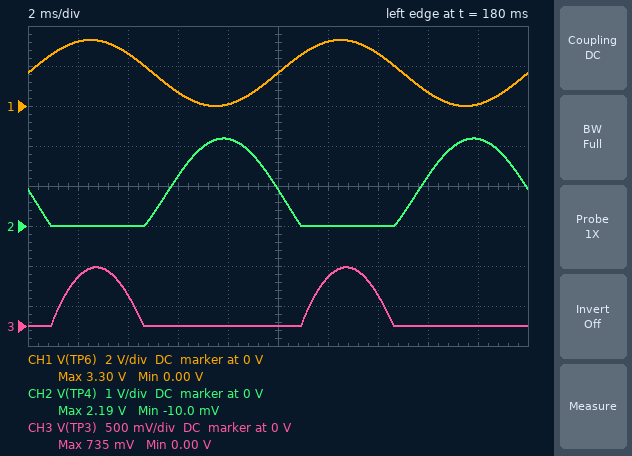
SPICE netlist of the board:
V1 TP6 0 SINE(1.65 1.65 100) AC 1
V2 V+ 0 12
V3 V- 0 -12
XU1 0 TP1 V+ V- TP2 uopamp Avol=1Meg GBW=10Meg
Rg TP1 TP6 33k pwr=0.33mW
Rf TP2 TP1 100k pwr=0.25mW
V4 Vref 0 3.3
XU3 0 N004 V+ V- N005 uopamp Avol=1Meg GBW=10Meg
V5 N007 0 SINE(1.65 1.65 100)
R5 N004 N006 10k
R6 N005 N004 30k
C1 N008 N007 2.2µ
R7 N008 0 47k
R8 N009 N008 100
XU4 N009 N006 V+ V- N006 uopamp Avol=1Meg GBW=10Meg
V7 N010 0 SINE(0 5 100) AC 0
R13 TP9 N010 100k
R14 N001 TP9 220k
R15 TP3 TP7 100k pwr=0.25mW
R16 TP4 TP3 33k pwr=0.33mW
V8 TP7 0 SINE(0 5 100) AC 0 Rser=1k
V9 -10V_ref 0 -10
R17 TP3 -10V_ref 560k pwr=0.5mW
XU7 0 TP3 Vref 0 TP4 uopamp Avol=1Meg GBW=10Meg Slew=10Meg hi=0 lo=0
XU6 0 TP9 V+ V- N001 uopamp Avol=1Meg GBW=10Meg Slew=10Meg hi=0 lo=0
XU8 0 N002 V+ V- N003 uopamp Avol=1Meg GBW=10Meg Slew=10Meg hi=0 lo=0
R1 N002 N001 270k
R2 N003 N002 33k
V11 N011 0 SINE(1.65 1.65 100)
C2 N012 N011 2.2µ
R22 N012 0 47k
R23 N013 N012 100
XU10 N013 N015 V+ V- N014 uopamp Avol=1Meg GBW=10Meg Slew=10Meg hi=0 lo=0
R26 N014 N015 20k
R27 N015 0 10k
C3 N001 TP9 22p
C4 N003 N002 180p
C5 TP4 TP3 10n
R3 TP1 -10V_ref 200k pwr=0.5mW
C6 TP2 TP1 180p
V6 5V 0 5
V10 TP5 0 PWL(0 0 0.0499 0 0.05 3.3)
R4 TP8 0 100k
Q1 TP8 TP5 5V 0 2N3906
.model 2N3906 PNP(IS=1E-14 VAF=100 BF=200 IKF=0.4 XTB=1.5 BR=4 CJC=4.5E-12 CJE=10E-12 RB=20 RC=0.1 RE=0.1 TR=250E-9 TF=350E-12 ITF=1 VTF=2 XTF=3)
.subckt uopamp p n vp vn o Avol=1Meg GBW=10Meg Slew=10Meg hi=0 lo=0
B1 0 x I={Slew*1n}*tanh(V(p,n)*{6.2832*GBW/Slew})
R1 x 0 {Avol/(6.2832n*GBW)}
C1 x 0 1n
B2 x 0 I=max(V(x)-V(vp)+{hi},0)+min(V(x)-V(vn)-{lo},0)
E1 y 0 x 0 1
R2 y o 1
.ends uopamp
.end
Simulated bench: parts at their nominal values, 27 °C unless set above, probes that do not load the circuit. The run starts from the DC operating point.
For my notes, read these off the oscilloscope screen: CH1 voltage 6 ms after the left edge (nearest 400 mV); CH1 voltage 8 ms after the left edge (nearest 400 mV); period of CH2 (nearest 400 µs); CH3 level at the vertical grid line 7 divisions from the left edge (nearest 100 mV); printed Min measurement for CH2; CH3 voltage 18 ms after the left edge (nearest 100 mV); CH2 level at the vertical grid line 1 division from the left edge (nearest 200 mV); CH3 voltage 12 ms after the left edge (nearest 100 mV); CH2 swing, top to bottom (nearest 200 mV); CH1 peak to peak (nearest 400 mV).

800 mV
0 V
10.0 ms
400 mV
-10.0 mV
0 V
0 V
600 mV
2.2 V
3.2 V
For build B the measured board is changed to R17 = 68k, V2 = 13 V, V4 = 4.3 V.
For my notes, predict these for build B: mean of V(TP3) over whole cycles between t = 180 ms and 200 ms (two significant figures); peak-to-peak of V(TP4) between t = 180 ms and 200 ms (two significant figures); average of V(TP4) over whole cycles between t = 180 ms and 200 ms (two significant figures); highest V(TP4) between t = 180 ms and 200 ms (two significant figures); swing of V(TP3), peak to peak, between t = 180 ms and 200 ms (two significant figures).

-450 mV
1.1 V
4.0 V
4.3 V
1.2 V
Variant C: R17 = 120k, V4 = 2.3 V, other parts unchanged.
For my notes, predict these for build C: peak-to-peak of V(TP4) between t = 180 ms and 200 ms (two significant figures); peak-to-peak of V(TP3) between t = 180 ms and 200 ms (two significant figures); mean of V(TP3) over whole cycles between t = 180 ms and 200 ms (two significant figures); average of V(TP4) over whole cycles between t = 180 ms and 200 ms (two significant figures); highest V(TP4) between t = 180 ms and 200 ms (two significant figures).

1.2 V
1.3 V
-470 mV
2.0 V
2.3 V
